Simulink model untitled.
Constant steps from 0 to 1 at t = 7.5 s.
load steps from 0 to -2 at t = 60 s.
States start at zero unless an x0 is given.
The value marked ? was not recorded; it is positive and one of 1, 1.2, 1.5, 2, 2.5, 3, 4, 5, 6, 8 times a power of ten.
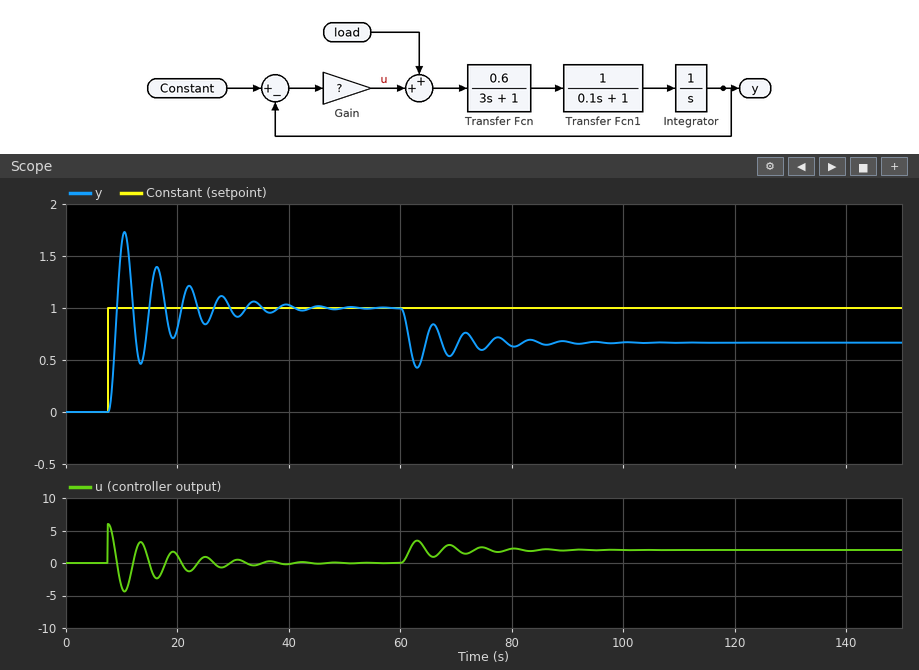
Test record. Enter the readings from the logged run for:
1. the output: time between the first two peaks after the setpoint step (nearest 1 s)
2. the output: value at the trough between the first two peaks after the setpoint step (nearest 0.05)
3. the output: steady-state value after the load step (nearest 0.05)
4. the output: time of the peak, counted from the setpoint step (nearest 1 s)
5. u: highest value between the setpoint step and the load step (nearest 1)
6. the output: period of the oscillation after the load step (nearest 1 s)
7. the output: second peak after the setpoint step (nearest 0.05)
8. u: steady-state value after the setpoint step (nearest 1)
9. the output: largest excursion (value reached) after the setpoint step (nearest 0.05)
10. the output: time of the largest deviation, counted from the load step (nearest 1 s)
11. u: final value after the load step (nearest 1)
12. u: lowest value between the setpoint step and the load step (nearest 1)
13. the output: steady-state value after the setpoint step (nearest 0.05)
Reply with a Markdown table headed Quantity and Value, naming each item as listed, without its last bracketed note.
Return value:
| Quantity | Value |
|---|---|
| the output: time between the first two peaks after the setpoint step | 6 s |
| the output: value at the trough between the first two peaks after the setpoint step | 0.45 |
| the output: steady-state value after the load step | 0.65 |
| the output: time of the peak, counted from the setpoint step | 3 s |
| u: highest value between the setpoint step and the load step | 6 |
| the output: period of the oscillation after the load step | 6 s |
| the output: second peak after the setpoint step | 1.40 |
| u: steady-state value after the setpoint step | 0 |
| the output: largest excursion (value reached) after the setpoint step | 1.75 |
| the output: time of the largest deviation, counted from the load step | 3 s |
| u: final value after the load step | 2 |
| u: lowest value between the setpoint step and the load step | -4 |
| the output: steady-state value after the setpoint step | 1.00 |
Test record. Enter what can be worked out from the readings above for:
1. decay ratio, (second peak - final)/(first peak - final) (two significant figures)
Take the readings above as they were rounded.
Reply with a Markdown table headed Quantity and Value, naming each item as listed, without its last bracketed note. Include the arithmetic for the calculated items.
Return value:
| Quantity | Value |
|---|---|
| decay ratio, (second peak - final)/(first peak - final) | (1.4 - 1) / (1.75 - 1) = 0.53 |
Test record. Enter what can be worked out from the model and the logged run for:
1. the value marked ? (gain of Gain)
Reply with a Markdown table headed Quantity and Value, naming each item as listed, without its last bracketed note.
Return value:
| Quantity | Value |
|---|---|
| the value marked ? | 6 |
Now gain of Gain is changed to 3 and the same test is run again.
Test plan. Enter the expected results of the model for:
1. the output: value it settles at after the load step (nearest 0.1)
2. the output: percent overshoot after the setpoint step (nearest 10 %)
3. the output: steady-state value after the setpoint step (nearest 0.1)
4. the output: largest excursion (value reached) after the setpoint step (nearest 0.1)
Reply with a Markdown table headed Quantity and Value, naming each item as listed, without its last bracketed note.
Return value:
| Quantity | Value |
|---|---|
| the output: value it settles at after the load step | 0.3 |
| the output: percent overshoot after the setpoint step | 60 % |
| the output: steady-state value after the setpoint step | 1.0 |
| the output: largest excursion (value reached) after the setpoint step | 1.6 |
